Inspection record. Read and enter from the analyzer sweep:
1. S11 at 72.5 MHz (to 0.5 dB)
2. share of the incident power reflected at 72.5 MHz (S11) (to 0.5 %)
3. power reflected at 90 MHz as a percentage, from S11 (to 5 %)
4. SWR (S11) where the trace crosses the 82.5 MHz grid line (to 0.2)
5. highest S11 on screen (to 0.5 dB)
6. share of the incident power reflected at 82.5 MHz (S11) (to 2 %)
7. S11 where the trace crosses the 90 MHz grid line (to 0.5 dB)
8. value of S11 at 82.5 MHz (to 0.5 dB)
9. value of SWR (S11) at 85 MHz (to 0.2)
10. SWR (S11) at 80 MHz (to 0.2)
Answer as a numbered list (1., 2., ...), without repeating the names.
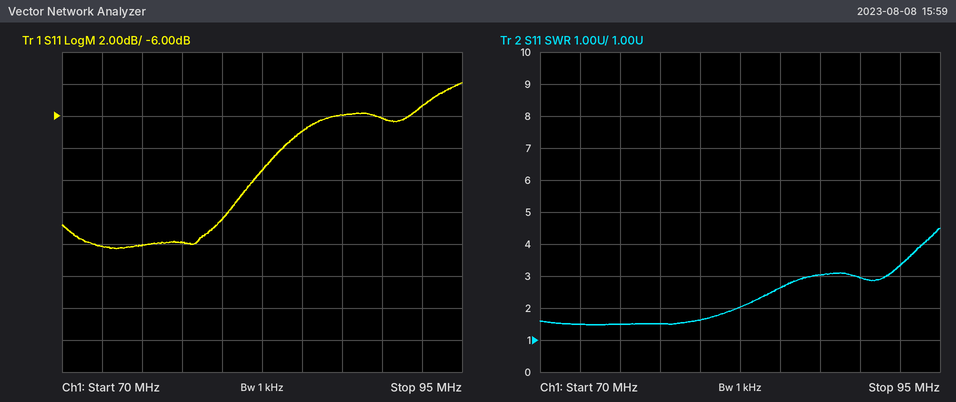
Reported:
1. -14.0 dB
2. 4.0 %
3. 25 %
4. 2.0
5. -4.0 dB
6. 12 %
7. -6.0 dB
8. -9.5 dB
9. 2.6
10. 1.6
